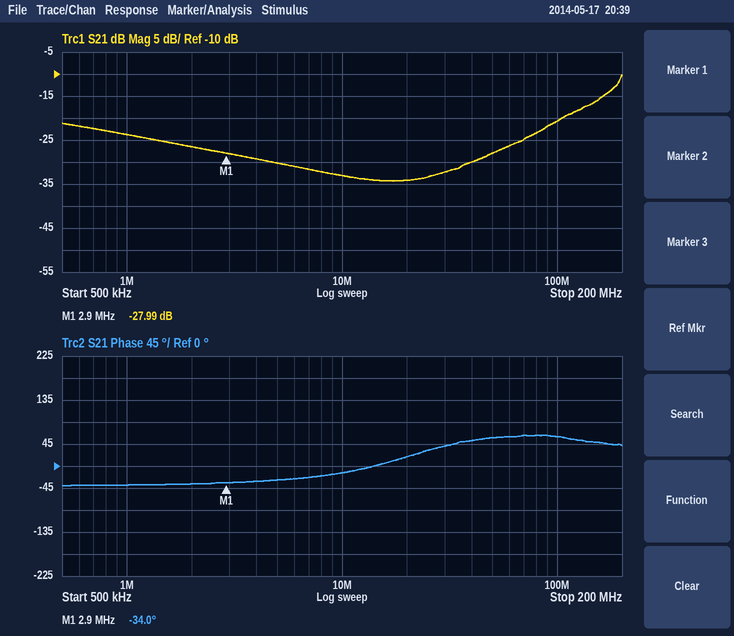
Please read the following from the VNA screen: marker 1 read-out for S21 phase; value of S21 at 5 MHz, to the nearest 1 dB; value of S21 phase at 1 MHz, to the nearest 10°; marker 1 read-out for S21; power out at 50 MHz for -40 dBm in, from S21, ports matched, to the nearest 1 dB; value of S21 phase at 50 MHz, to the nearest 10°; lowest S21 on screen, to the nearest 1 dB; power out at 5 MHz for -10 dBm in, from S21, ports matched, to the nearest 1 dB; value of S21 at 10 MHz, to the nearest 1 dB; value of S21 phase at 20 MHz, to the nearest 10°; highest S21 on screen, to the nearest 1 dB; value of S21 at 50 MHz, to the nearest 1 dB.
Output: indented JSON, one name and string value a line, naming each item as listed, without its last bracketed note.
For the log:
{
  "marker 1 read-out for S21 phase": "-34.0°",
  "value of S21 at 5 MHz, to the nearest 1 dB": "-30 dB",
  "value of S21 phase at 1 MHz, to the nearest 10°": "-40°",
  "marker 1 read-out for S21": "-27.99 dB",
  "power out at 50 MHz for -40 dBm in, from S21, ports matched, to the nearest 1 dB": "-68 dBm",
  "value of S21 phase at 50 MHz, to the nearest 10°": "60°",
  "lowest S21 on screen, to the nearest 1 dB": "-34 dB",
  "power out at 5 MHz for -10 dBm in, from S21, ports matched, to the nearest 1 dB": "-40 dBm",
  "value of S21 at 10 MHz, to the nearest 1 dB": "-33 dB",
  "value of S21 phase at 20 MHz, to the nearest 10°": "20°",
  "highest S21 on screen, to the nearest 1 dB": "-10 dB",
  "value of S21 at 50 MHz, to the nearest 1 dB": "-28 dB"
}
